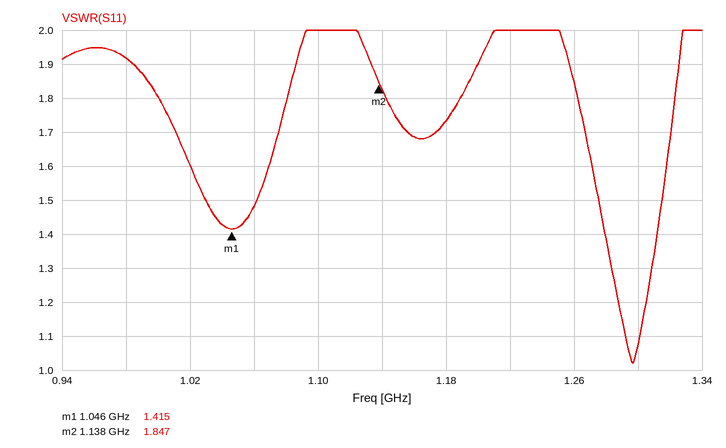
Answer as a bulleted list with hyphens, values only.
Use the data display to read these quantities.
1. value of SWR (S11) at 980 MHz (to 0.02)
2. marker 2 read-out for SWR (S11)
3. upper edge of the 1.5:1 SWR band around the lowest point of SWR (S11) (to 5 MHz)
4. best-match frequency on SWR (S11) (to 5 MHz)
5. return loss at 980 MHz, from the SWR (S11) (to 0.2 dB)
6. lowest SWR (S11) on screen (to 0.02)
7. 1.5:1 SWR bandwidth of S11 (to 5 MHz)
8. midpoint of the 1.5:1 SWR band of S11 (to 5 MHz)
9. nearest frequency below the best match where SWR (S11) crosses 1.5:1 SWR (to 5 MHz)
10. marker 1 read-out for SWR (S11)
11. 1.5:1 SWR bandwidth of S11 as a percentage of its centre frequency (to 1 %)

- 1.92
- 1.847
- 1.315 GHz
- 1.295 GHz
- 10.0 dB
- 1.02
- 40 MHz
- 1.295 GHz
- 1.275 GHz
- 1.415
- 3 %
